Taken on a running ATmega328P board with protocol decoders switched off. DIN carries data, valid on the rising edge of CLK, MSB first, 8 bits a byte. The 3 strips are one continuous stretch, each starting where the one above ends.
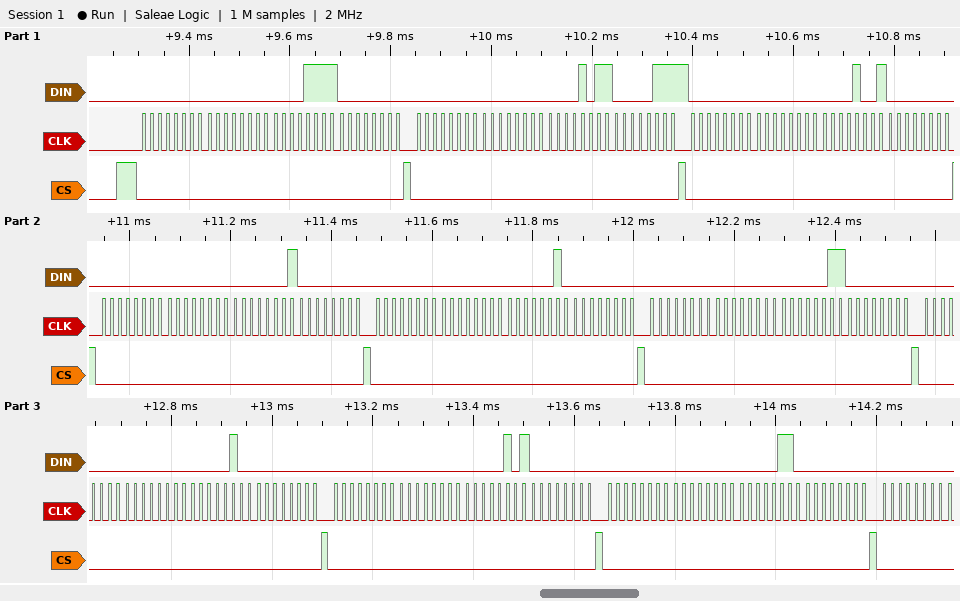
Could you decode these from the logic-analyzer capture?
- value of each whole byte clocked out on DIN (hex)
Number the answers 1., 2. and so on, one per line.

1. 00 00 0F 00 00 00 0B 07 00 00 09 00 00 00 01 00 00 00 02 00 00 00 03 00 00 00 04 00 00 00 05 00 00 00 06 00 00
